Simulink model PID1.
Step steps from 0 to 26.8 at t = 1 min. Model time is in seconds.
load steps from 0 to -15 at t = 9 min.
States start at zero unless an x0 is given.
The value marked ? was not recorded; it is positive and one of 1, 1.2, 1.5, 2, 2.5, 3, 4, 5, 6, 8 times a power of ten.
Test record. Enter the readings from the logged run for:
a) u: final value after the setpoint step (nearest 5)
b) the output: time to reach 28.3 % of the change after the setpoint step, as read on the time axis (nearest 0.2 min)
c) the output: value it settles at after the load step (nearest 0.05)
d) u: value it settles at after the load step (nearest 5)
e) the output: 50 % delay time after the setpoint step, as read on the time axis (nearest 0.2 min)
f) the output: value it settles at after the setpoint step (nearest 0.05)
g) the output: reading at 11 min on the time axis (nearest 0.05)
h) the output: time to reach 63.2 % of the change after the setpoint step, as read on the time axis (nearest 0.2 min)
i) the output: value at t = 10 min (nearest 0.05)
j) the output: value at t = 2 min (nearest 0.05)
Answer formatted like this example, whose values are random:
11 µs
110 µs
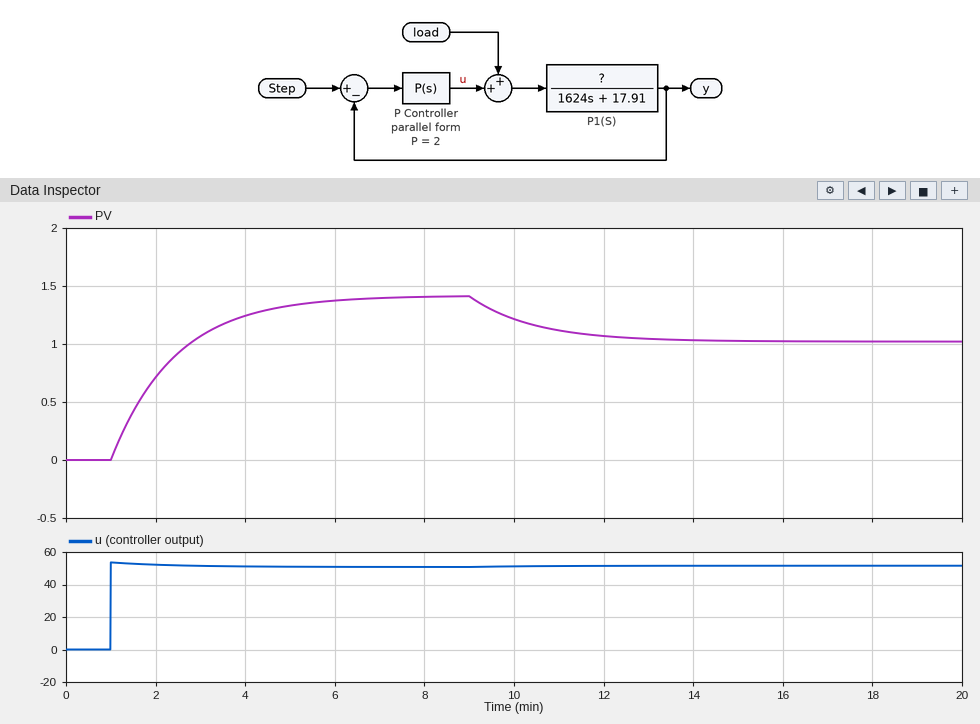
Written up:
50
1.4 min
1.00
50
2.0 min
1.40
1.10
2.4 min
1.20
0.70
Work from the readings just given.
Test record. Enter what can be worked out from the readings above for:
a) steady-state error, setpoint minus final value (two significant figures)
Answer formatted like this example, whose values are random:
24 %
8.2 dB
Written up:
25
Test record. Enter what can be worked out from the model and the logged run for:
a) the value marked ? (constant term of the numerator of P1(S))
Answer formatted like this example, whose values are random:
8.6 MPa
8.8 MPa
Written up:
0.5
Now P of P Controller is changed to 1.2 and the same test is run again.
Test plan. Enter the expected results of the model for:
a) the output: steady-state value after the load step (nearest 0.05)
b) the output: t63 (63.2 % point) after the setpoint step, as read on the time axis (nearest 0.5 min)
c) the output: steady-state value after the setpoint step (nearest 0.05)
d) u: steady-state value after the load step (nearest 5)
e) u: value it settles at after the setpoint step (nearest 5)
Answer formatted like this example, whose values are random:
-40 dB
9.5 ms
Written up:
0.45
2.5 min
0.85
30
30
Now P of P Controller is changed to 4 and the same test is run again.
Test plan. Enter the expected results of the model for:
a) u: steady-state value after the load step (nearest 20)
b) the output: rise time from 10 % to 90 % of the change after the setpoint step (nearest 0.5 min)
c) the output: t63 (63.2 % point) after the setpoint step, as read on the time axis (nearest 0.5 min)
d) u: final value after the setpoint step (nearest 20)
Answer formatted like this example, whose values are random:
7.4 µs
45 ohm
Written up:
100
3.0 min
2.5 min
100
